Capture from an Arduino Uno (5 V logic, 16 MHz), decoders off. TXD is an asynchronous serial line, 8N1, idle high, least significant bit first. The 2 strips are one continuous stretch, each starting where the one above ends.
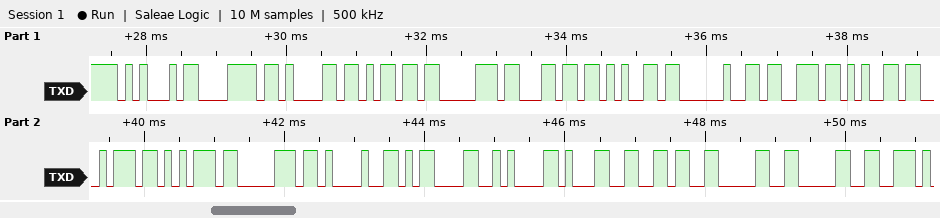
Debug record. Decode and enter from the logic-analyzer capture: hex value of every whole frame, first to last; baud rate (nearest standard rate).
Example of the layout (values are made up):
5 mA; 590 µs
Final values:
45 78 61 6D 70 6C 65 20 73 65 74 75 70 21 0D 0A 31 36 30 30; 9600 baud
